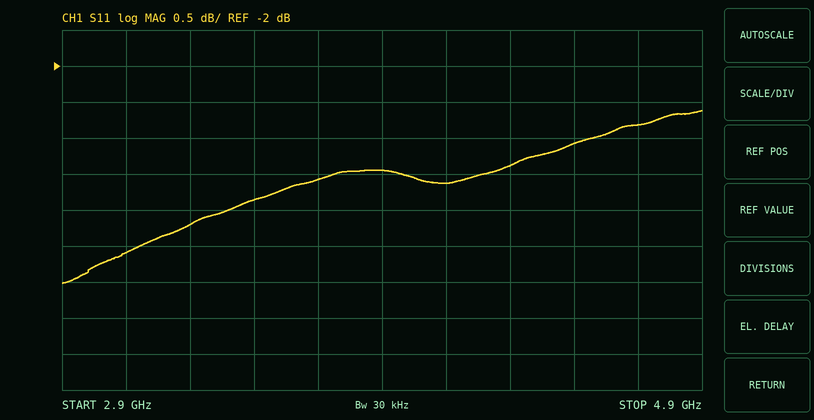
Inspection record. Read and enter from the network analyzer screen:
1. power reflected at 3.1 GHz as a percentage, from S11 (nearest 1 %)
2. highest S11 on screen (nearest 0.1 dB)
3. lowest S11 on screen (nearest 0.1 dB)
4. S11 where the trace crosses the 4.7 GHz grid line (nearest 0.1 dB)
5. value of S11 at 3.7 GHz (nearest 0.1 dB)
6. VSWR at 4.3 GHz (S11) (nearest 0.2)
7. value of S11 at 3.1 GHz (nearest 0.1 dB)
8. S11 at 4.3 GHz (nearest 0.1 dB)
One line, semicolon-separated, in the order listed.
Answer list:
35 %; -2.6 dB; -5.0 dB; -2.8 dB; -3.6 dB; 5.2; -4.6 dB; -3.4 dB
